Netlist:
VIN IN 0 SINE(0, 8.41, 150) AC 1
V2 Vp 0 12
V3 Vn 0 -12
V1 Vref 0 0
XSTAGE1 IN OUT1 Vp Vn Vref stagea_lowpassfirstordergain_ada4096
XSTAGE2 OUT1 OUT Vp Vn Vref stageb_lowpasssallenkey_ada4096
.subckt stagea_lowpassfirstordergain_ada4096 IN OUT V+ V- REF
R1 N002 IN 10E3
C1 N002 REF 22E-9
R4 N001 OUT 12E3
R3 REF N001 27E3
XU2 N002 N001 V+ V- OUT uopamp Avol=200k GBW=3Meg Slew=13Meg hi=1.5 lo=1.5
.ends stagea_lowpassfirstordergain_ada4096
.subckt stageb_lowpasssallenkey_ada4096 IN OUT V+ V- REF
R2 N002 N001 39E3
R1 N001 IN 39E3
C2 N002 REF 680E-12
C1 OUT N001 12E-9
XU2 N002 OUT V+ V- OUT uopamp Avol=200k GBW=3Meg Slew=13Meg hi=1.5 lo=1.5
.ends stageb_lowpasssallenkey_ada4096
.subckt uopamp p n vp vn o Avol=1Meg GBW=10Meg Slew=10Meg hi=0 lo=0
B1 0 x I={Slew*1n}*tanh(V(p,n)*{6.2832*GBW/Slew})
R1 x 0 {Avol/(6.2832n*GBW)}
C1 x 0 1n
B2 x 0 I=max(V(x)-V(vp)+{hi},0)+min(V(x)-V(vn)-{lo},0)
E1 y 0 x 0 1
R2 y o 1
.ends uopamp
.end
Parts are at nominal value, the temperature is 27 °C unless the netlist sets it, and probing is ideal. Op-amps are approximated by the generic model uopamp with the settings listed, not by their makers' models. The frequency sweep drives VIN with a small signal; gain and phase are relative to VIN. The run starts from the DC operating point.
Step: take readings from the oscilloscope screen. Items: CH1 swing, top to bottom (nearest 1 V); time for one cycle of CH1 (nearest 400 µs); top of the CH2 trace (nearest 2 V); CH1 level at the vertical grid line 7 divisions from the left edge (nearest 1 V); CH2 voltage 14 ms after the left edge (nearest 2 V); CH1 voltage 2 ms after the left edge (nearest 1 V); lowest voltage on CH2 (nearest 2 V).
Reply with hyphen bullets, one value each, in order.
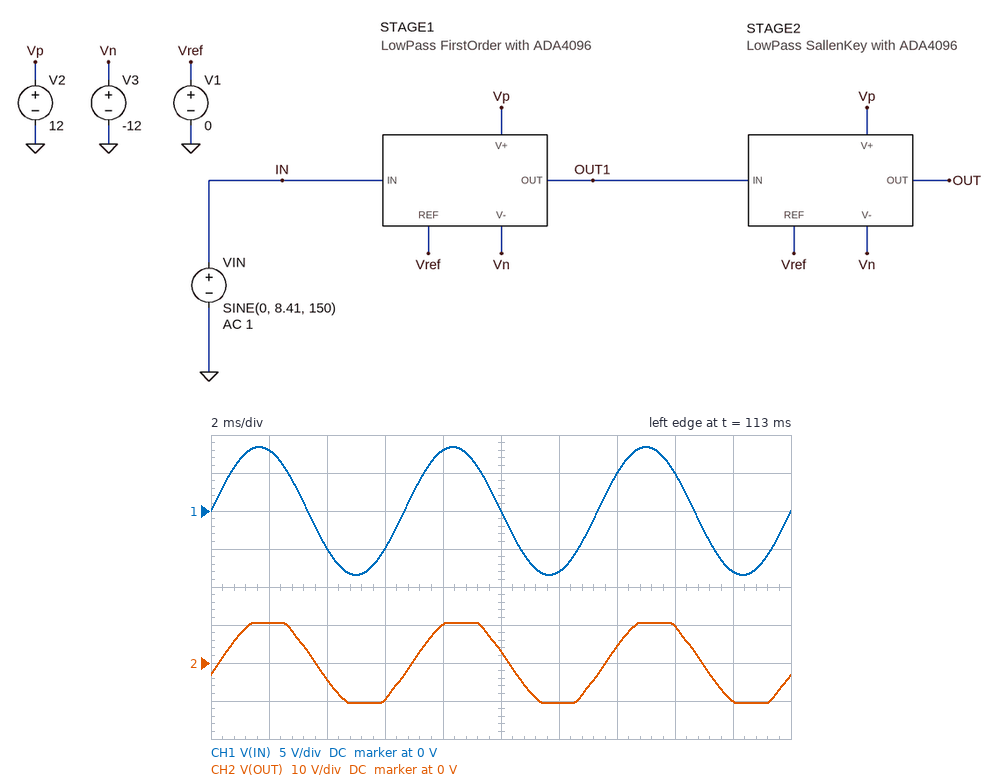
- 17 V
- 6.8 ms
- 10 V
- 5 V
- 4 V
- 8 V
- -10 V
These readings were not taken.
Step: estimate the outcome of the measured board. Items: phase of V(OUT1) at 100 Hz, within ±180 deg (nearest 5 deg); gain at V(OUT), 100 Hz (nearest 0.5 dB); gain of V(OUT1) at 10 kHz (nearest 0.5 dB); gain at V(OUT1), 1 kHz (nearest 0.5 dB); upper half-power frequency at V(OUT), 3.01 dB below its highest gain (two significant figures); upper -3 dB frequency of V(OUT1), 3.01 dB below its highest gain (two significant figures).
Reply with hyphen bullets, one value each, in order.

- -10 deg
- 3.0 dB
- -19.5 dB
- -1.5 dB
- 1.6 kHz
- 720 Hz
